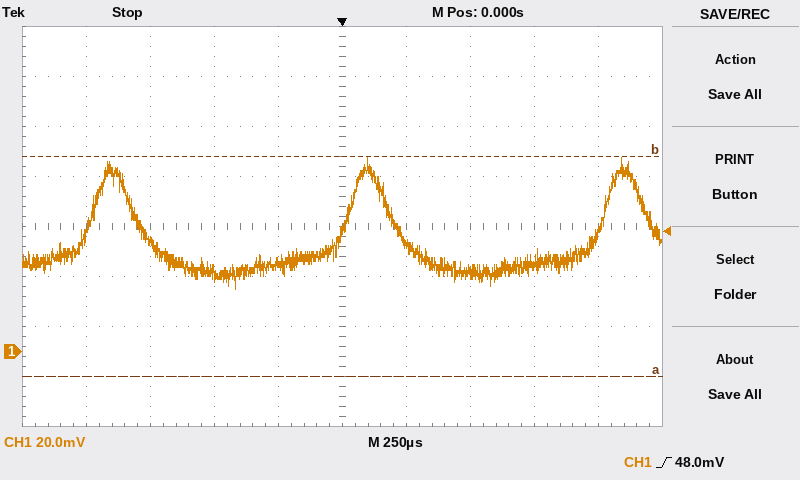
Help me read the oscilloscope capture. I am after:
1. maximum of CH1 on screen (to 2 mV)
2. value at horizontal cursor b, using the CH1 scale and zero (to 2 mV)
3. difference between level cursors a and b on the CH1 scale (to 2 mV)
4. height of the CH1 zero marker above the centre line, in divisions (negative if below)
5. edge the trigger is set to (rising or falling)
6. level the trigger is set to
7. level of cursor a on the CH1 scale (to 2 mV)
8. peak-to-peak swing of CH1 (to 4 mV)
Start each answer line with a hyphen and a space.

- 78 mV
- 78 mV
- 88 mV
- -2.5 div
- rising
- 48.0 mV
- -10 mV
- 52 mV
